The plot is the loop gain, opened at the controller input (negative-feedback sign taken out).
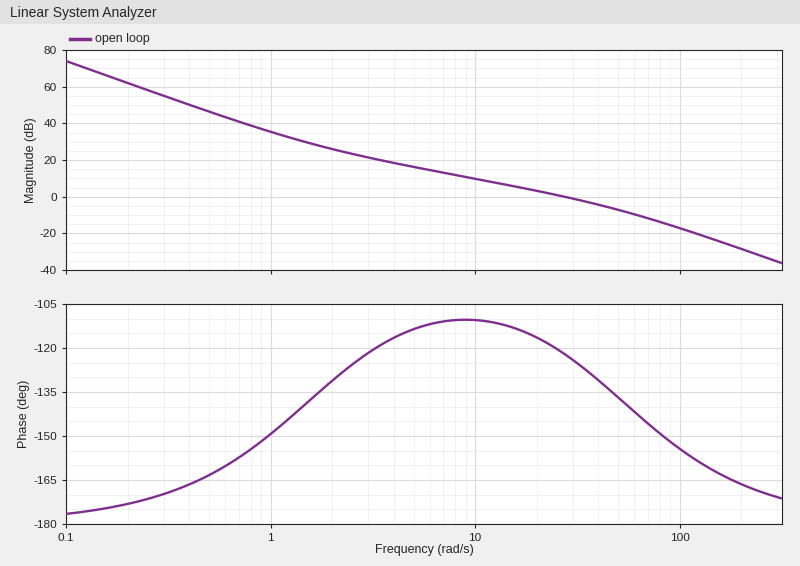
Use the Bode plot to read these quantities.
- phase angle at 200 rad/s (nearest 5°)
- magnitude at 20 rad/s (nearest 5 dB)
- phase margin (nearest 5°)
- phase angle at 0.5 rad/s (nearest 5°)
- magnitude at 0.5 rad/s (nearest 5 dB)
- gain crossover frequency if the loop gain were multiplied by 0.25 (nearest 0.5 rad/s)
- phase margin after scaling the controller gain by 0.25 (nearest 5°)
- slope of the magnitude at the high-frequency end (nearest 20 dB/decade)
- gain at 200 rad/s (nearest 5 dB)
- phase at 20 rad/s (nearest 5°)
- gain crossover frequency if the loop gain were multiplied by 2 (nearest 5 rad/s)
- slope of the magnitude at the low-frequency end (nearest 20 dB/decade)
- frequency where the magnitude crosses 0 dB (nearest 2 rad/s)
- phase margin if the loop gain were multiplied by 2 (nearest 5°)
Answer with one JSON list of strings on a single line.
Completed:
["-165°", "5 dB", "60°", "-165°", "45 dB", "8.0 rad/s", "70°", "-40 dB/decade", "-30 dB", "-115°", "45 rad/s", "-40 dB/decade", "28 rad/s", "45°"]
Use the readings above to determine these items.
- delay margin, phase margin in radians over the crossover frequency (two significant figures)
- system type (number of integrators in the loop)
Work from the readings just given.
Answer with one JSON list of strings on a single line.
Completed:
["0.037 s", "2"]
